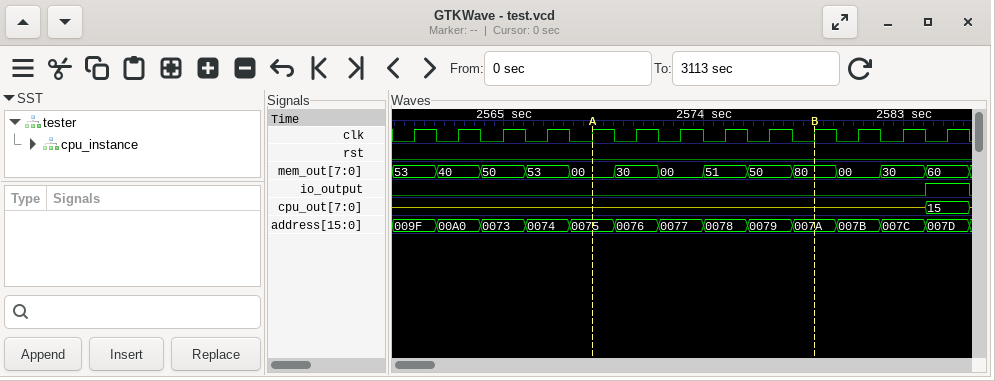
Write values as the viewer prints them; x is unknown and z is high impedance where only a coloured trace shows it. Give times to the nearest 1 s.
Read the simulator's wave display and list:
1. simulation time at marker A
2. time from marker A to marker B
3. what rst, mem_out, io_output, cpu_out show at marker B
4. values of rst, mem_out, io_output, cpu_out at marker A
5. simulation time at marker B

2569 s
10 s
rst=0, mem_out=80, io_output=0, cpu_out=z
rst=0, mem_out=00, io_output=0, cpu_out=z
2579 s
